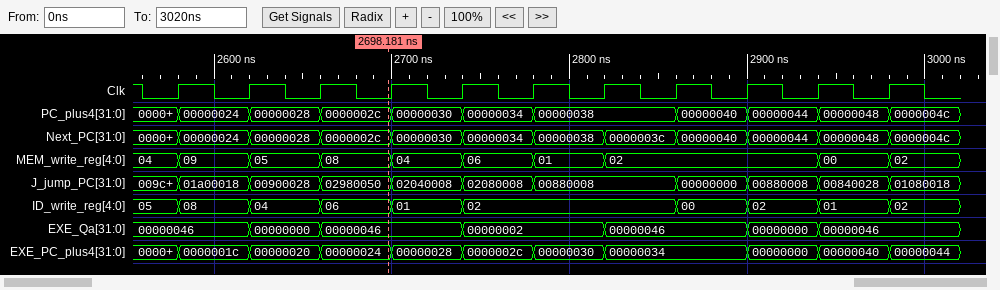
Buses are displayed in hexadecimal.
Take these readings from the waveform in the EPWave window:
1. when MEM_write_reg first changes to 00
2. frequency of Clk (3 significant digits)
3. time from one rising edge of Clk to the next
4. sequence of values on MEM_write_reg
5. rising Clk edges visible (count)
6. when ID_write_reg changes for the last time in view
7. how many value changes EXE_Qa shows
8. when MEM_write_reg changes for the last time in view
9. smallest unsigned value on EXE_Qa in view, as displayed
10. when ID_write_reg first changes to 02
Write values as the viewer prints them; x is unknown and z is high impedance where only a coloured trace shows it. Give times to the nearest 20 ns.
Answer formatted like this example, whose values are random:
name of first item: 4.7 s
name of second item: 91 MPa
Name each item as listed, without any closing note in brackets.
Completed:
when MEM_write_reg first changes to 00: 2940 ns
frequency of Clk: 25.0 MHz
time from one rising edge of Clk to the next: 40 ns
sequence of values on MEM_write_reg: 04, 09, 05, 08, 04, 06, 01, 02, 00, 02
rising Clk edges visible: 11
when ID_write_reg changes for the last time in view: 2980 ns
how many value changes EXE_Qa shows: 6
when MEM_write_reg changes for the last time in view: 2980 ns
smallest unsigned value on EXE_Qa in view, as displayed: 00000000
when ID_write_reg first changes to 02: 2740 ns
